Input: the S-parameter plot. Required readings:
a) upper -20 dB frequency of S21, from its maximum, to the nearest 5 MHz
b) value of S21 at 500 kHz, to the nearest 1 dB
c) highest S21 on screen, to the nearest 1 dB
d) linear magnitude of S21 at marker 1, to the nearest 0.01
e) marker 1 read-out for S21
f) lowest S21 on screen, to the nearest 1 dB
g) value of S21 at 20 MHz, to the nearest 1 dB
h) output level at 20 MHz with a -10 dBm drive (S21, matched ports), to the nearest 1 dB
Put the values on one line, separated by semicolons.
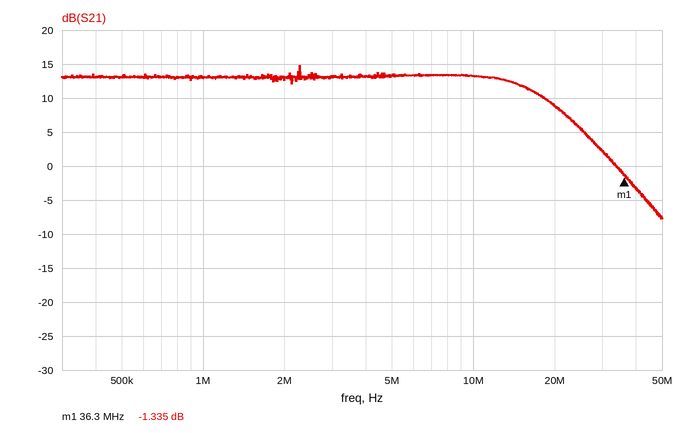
45 MHz; 13 dB; 15 dB; 0.86; -1.335 dB; -8 dB; 9 dB; -1 dBm
